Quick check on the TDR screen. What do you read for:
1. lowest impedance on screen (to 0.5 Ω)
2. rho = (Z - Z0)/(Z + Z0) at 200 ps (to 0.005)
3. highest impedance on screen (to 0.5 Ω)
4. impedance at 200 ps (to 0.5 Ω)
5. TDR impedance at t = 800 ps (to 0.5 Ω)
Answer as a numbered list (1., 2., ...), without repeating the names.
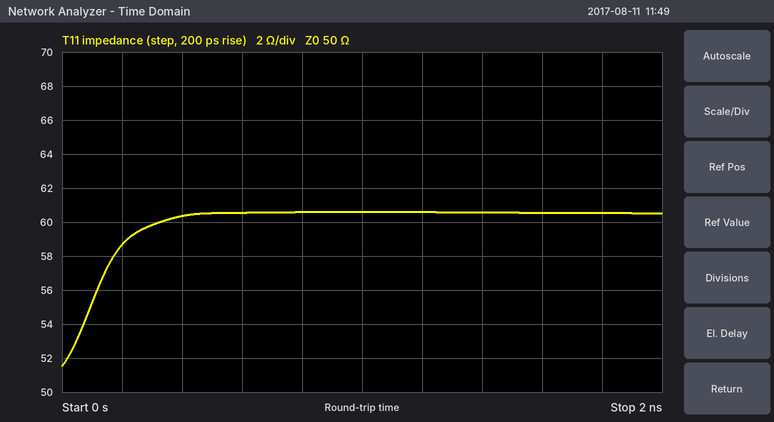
1. 51.5 Ω
2. +0.080
3. 60.5 Ω
4. 58.5 Ω
5. 60.5 Ω
